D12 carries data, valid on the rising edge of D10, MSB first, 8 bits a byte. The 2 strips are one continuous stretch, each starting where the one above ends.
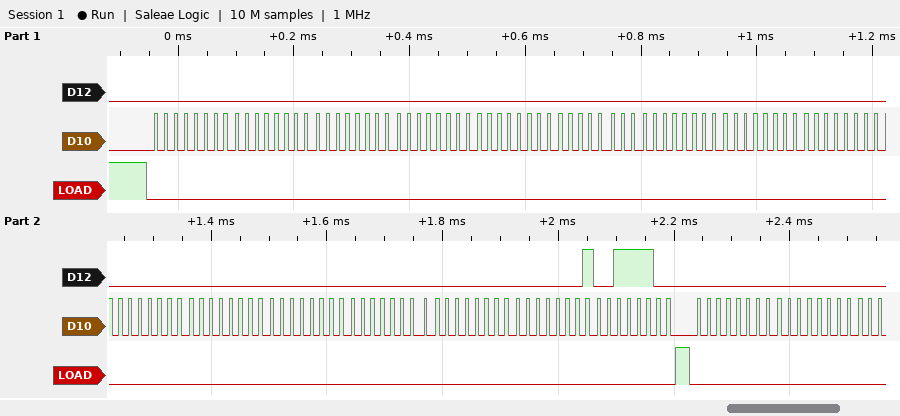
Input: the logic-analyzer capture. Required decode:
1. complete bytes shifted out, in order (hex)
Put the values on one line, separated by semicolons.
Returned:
00 00 00 00 00 00 00 00 00 00 00 00 00 00 01 3C 00 00
